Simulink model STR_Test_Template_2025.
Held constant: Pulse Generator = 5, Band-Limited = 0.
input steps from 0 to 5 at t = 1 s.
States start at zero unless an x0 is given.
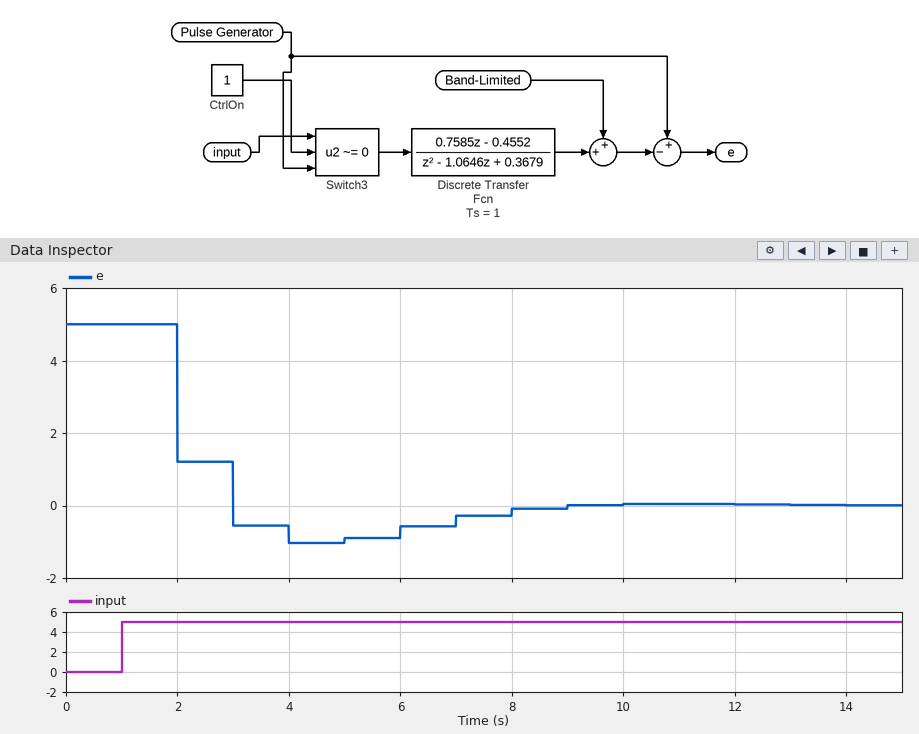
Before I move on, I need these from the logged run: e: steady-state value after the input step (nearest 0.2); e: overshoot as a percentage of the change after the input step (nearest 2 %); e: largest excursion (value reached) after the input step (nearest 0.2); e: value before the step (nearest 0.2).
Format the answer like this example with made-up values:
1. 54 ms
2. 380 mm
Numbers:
1. 0.0
2. 20 %
3. -1.0
4. 5.0
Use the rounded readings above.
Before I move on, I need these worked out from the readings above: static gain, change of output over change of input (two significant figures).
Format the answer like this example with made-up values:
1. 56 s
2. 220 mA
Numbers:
1. -1.0
